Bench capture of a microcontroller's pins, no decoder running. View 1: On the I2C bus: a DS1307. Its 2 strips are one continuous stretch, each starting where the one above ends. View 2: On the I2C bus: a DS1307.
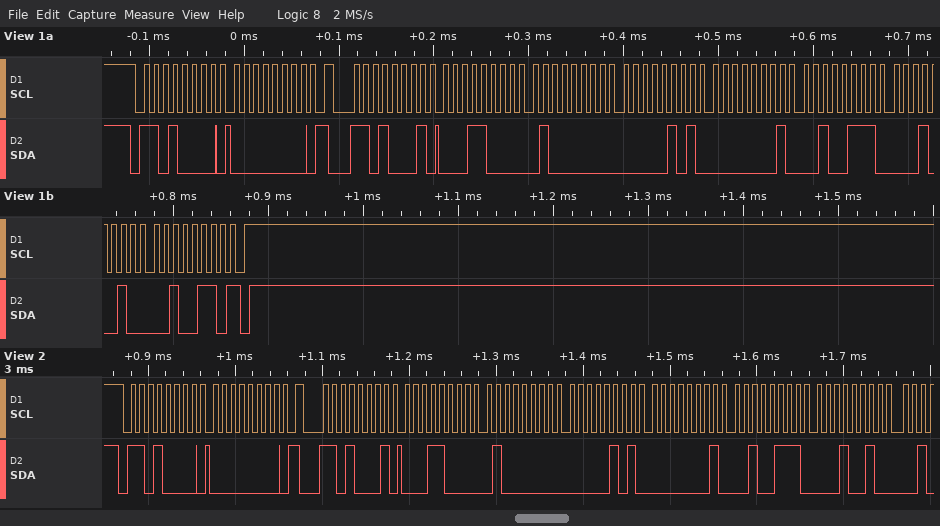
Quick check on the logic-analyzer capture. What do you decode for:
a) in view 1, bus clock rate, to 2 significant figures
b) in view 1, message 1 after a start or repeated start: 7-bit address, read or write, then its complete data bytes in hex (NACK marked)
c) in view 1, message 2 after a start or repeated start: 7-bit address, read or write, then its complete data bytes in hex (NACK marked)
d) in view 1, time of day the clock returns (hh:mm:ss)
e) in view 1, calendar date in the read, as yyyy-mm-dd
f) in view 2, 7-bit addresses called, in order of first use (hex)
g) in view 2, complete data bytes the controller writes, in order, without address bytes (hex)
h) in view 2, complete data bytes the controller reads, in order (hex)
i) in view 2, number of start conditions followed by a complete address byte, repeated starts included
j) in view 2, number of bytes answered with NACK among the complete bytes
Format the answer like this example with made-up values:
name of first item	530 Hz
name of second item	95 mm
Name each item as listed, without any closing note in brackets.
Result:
in view 1, bus clock rate, to 2 significant figures	100 kHz
in view 1, message 1 after a start or repeated start: 7-bit address, read or write, then its complete data bytes in hex	0x68 write: 00
in view 1, message 2 after a start or repeated start: 7-bit address, read or write, then its complete data bytes in hex	0x68 read: 18 40 05 01 27 12 26 NACK
in view 1, time of day the clock returns	05:40:18
in view 1, calendar date in the read, as yyyy-mm-dd	2026-12-27
in view 2, 7-bit addresses called, in order of first use	0x68
in view 2, complete data bytes the controller writes, in order, without address bytes	00
in view 2, complete data bytes the controller reads, in order	18 40 05 01 27 12
in view 2, number of start conditions followed by a complete address byte, repeated starts included	2
in view 2, number of bytes answered with NACK among the complete bytes	0
